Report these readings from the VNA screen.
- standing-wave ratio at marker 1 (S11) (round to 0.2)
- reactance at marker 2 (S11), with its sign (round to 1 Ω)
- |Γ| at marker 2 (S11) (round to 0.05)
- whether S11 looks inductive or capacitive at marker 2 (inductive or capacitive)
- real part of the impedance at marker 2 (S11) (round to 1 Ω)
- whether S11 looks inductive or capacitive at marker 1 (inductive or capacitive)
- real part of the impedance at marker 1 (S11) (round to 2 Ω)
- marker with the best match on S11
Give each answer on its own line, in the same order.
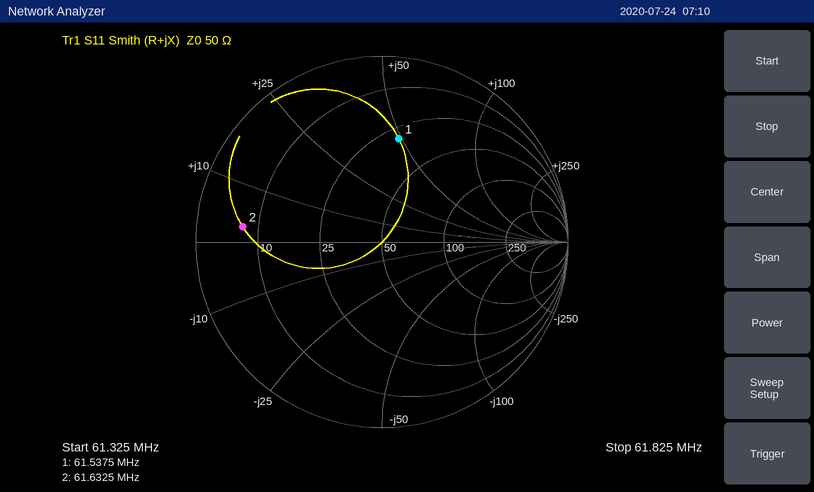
3.6
+3 Ω
0.75
inductive
7 Ω
inductive
30 Ω
marker 1
